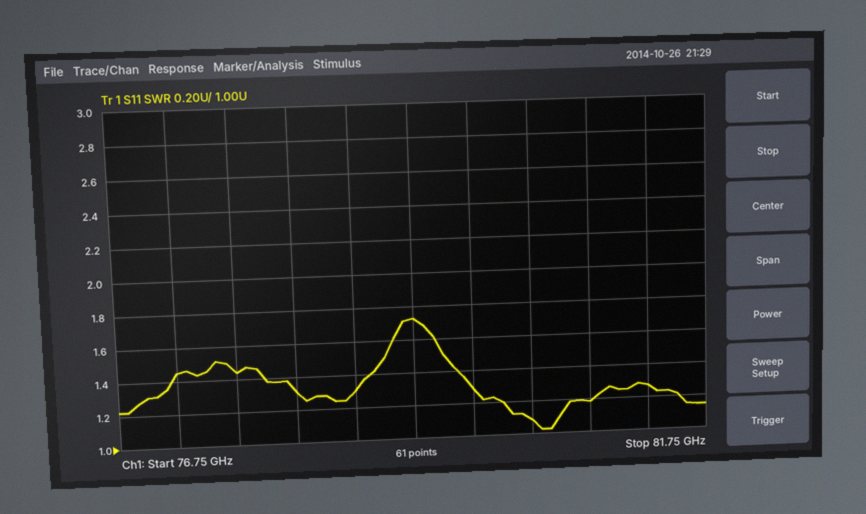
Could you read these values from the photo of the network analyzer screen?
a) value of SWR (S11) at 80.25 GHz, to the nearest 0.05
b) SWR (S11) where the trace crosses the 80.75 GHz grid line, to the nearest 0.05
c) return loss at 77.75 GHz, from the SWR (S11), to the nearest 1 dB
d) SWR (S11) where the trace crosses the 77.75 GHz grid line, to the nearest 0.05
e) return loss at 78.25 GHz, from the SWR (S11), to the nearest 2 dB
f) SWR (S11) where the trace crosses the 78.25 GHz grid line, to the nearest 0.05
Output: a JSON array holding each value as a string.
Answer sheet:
["1.10", "1.20", "15 dB", "1.45", "18 dB", "1.30"]
